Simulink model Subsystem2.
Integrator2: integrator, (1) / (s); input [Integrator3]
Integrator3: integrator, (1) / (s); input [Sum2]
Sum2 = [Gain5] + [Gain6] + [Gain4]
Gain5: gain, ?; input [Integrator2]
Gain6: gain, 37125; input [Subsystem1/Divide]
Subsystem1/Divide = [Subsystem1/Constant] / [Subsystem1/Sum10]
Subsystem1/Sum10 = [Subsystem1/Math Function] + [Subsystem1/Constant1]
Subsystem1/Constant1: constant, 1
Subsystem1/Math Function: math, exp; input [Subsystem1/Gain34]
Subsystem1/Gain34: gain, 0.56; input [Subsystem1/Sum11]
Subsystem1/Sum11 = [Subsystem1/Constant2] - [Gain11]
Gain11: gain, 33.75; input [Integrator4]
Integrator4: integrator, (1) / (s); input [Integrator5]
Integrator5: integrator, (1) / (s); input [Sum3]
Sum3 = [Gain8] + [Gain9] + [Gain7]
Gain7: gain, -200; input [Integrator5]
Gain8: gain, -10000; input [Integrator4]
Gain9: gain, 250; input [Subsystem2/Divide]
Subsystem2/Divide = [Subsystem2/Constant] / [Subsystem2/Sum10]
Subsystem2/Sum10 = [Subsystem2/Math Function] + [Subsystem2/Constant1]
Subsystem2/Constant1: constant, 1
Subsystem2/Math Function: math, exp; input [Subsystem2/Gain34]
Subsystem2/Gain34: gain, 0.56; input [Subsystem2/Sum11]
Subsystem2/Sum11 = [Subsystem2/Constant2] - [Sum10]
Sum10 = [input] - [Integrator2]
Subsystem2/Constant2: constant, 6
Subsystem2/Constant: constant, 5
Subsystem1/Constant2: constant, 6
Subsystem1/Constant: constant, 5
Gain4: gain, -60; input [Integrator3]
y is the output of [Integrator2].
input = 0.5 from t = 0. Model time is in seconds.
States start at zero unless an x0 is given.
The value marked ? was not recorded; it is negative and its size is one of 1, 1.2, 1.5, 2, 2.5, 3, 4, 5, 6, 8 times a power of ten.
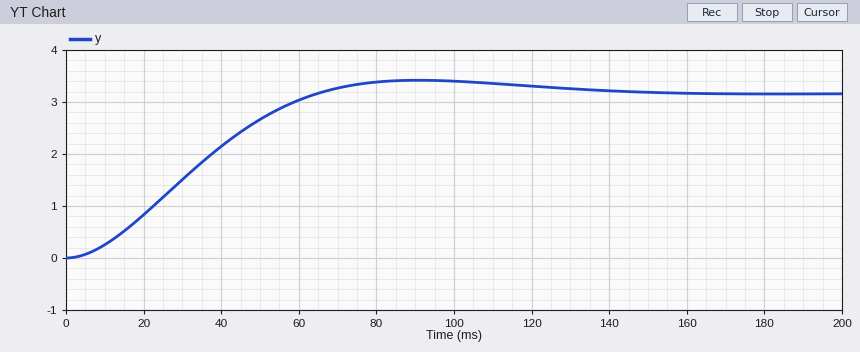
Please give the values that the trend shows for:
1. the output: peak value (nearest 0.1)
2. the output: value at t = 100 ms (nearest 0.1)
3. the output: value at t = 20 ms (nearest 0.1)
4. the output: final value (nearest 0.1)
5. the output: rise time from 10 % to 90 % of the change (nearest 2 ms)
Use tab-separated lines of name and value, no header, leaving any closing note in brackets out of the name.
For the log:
the output: peak value	3.4
the output: value at t = 100 ms	3.4
the output: value at t = 20 ms	0.8
the output: final value	3.2
the output: rise time from 10 % to 90 % of the change	44 ms
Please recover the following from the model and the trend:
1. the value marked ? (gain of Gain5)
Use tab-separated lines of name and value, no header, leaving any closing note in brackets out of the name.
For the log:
the value marked ?	-2000
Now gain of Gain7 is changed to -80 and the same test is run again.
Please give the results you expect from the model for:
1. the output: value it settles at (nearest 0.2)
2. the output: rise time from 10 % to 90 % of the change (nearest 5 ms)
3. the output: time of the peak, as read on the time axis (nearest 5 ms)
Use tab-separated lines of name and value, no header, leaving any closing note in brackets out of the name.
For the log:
the output: value it settles at	3.2
the output: rise time from 10 % to 90 % of the change	40 ms
the output: time of the peak, as read on the time axis	90 ms
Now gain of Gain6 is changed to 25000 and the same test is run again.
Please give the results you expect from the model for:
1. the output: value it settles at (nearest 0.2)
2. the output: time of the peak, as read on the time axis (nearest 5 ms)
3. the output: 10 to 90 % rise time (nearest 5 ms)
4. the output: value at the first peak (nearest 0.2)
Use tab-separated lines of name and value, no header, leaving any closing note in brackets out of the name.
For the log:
the output: value it settles at	2.2
the output: time of the peak, as read on the time axis	90 ms
the output: 10 to 90 % rise time	45 ms
the output: value at the first peak	2.4
